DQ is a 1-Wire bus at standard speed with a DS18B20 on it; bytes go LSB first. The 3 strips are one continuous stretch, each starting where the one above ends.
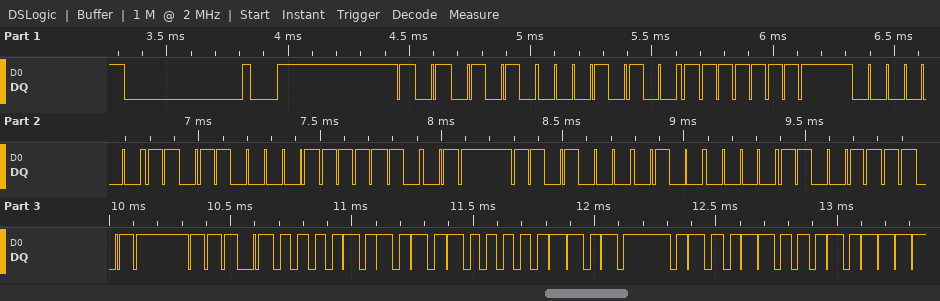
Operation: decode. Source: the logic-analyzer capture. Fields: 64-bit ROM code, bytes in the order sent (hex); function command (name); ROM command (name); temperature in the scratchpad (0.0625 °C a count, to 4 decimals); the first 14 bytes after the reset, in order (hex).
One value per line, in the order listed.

28 FF C0 86 9F 17 02 F3
Read Scratchpad
Match ROM
85.0000 °C
55 28 FF C0 86 9F 17 02 F3 BE 50 05 4B 46
